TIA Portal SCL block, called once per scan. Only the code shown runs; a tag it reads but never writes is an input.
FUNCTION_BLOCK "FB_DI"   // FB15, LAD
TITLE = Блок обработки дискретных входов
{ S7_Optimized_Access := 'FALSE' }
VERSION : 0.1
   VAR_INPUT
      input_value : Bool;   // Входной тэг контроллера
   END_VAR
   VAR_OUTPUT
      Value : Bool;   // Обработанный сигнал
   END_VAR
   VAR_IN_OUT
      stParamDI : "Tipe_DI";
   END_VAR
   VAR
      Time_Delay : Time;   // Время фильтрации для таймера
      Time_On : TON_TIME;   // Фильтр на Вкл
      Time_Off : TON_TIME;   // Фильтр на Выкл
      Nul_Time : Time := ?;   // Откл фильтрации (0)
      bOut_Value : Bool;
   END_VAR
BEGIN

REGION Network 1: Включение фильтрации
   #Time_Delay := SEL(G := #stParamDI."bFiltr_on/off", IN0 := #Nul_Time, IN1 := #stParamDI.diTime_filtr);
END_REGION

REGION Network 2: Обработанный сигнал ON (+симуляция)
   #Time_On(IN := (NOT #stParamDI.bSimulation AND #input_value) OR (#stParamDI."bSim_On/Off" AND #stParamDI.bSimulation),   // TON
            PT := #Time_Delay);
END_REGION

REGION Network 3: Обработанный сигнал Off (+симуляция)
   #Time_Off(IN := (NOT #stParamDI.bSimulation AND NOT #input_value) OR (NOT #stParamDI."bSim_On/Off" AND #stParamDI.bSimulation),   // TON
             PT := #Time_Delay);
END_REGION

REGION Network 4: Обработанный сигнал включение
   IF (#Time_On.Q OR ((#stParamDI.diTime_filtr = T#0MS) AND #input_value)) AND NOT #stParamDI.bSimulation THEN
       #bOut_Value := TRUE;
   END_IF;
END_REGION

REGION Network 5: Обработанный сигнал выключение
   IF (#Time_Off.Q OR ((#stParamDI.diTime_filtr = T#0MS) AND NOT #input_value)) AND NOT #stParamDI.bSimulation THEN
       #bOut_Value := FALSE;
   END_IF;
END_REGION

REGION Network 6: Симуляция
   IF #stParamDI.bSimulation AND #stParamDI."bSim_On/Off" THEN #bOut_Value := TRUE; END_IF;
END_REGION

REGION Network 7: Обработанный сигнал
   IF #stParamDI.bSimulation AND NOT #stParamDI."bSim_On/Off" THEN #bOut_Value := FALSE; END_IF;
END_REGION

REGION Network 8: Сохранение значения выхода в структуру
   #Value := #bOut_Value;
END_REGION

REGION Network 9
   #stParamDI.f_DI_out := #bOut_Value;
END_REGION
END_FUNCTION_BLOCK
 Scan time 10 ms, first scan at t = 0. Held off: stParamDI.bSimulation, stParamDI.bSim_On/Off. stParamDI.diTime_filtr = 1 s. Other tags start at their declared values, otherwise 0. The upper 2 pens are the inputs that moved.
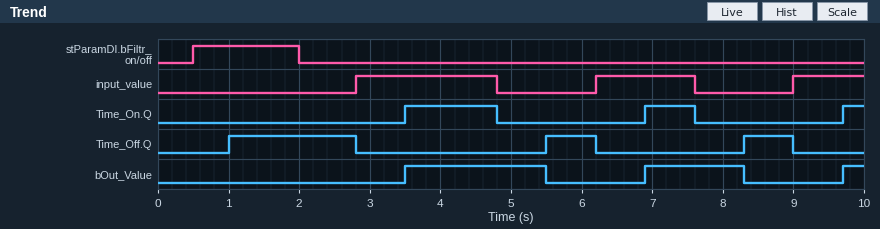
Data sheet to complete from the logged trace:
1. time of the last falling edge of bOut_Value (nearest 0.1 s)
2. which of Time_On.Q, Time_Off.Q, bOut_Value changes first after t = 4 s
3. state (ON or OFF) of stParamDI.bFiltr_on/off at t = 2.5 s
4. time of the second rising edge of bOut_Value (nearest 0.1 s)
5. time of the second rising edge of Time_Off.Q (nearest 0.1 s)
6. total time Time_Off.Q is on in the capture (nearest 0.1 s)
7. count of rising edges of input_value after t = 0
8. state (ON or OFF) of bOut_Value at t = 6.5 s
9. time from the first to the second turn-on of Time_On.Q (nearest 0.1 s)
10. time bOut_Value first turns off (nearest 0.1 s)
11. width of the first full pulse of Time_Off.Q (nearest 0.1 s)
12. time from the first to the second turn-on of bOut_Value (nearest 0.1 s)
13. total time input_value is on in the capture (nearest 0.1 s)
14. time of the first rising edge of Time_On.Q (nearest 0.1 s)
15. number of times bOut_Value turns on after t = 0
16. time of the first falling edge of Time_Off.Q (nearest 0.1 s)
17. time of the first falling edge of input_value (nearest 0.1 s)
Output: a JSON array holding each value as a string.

["8.3 s", "Time_On.Q", "OFF", "6.9 s", "5.5 s", "3.2 s", "3", "OFF", "3.4 s", "5.5 s", "1.8 s", "3.4 s", "4.4 s", "3.5 s", "3", "2.8 s", "4.8 s"]
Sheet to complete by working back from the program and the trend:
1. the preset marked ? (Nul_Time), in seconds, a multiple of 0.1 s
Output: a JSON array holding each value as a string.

["0.7 s"]
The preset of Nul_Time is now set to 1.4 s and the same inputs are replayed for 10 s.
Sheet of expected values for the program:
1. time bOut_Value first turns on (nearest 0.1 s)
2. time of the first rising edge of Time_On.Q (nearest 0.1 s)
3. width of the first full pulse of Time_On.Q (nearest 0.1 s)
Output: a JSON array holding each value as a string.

["4.2 s", "4.2 s", "0.6 s"]
